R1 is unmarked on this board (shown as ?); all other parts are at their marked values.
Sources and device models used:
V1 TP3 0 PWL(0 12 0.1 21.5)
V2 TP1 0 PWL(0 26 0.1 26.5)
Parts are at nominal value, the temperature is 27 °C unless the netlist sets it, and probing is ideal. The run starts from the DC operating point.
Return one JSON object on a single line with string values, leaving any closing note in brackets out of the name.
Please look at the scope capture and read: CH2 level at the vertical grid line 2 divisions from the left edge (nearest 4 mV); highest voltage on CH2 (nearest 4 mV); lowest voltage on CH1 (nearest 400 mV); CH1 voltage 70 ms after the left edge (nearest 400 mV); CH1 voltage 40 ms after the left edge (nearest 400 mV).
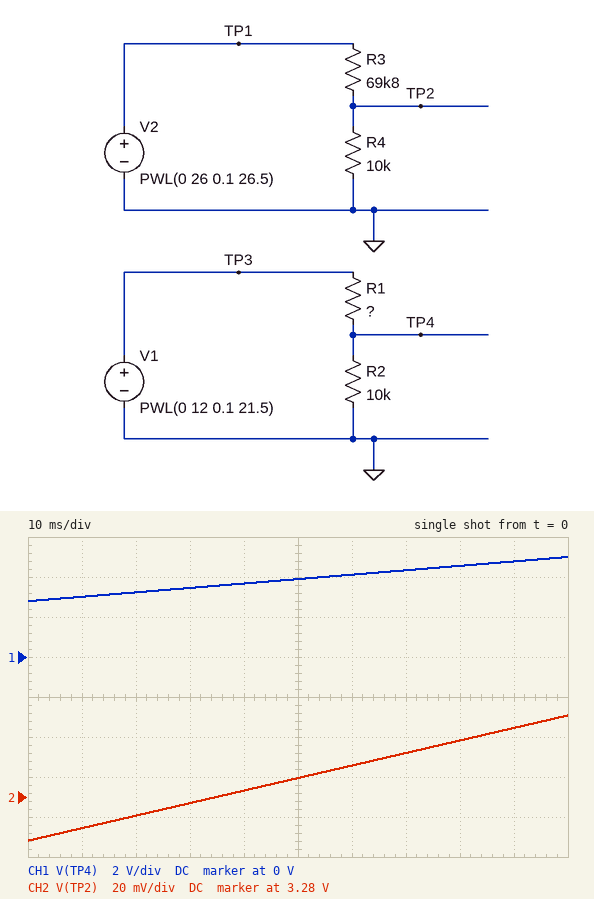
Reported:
{"CH2 level at the vertical grid line 2 divisions from the left edge": "3.272 V", "highest voltage on CH2": "3.320 V", "lowest voltage on CH1": "2.8 V", "CH1 voltage 70 ms after the left edge": "4.4 V", "CH1 voltage 40 ms after the left edge": "3.6 V"}
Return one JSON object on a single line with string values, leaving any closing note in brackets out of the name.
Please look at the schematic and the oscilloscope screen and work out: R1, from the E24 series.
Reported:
{"R1, from the E24 series": "33 kΩ"}
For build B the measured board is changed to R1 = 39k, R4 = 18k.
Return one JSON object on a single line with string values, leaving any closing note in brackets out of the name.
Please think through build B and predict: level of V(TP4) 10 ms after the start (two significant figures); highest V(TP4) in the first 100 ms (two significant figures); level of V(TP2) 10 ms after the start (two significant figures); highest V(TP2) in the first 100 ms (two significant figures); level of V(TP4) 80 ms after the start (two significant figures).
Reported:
{"level of V(TP4) 10 ms after the start": "2.6 V", "highest V(TP4) in the first 100 ms": "4.4 V", "level of V(TP2) 10 ms after the start": "5.3 V", "highest V(TP2) in the first 100 ms": "5.4 V", "level of V(TP4) 80 ms after the start": "4.0 V"}
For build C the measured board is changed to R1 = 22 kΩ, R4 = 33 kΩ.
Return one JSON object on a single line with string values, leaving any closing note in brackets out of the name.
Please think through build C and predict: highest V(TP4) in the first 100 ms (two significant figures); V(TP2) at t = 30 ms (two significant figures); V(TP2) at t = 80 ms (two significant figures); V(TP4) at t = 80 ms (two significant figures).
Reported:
{"highest V(TP4) in the first 100 ms": "6.7 V", "V(TP2) at t = 30 ms": "8.4 V", "V(TP2) at t = 80 ms": "8.5 V", "V(TP4) at t = 80 ms": "6.1 V"}
